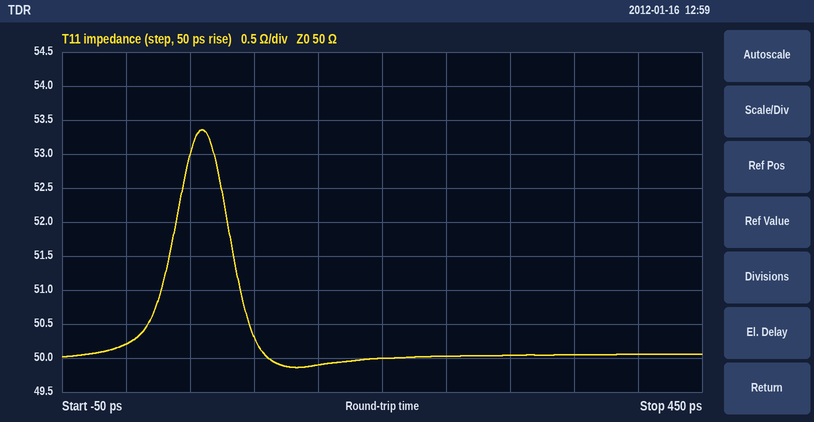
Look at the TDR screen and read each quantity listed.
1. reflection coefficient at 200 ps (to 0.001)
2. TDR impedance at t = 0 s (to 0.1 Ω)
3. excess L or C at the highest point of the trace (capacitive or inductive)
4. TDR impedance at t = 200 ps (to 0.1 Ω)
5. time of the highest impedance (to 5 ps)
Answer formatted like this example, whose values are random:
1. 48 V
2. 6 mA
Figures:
1. 0.000
2. 50.2 Ω
3. inductive
4. 50.0 Ω
5. 60 ps
